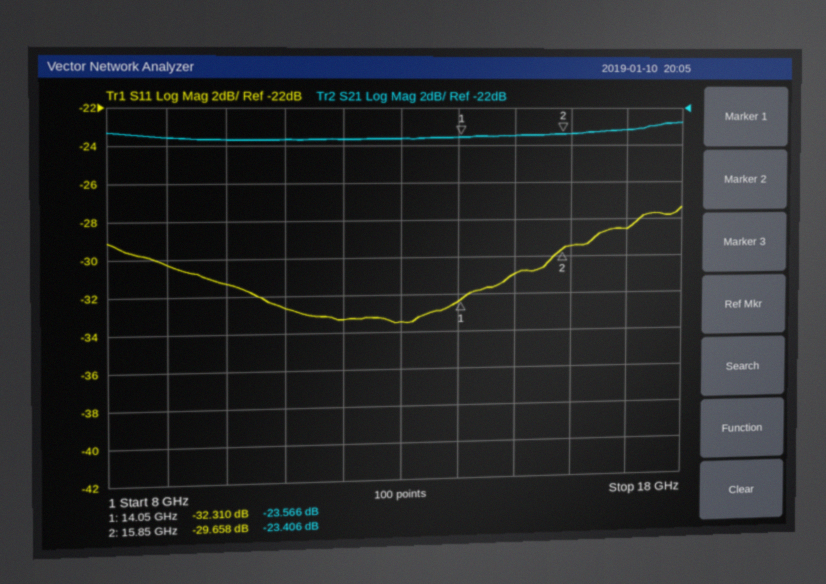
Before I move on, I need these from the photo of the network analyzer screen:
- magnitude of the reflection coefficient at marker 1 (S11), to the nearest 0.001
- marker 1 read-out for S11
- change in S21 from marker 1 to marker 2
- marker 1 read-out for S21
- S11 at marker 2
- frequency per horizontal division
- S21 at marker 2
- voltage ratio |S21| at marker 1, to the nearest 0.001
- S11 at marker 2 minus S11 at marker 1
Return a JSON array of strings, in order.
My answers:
["0.024", "-32.310 dB", "0.160 dB", "-23.566 dB", "-29.658 dB", "1 GHz", "-23.406 dB", "0.066", "2.652 dB"]
